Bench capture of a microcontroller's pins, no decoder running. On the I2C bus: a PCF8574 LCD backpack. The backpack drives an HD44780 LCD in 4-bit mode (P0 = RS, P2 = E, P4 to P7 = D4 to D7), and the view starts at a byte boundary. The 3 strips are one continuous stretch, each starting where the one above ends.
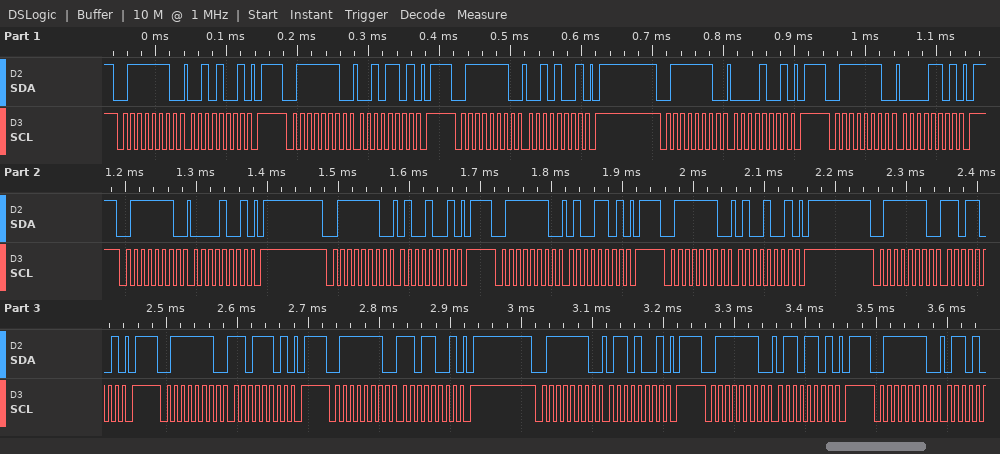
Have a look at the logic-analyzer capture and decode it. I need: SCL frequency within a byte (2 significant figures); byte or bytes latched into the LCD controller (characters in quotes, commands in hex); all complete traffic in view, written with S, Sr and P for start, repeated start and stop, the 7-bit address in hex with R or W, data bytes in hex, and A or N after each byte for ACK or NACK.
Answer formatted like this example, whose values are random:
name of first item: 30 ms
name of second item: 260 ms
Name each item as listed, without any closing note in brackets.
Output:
SCL frequency within a byte: 100 kHz
byte or bytes latched into the LCD controller: ' ' 'M'
all complete traffic in view, written with S, Sr and P for start, repeated start and stop, the 7-bit address in hex with R or W, data bytes in hex, and A or N after each byte for ACK or NACK: S 3FW A 29 A P S 3FW A 2D A P S 3FW A 29 A P S 3FW A 09 A P S 3FW A 0D A P S 3FW A 09 A P S 3FW A 49 A P S 3FW A 4D A P S 3FW A 49 A P S 3FW A D9 A P S 3FW A DD A P S 3FW A D9 A P S 3FW A 69 A P S 3FW A 6D A P S 3FW A
